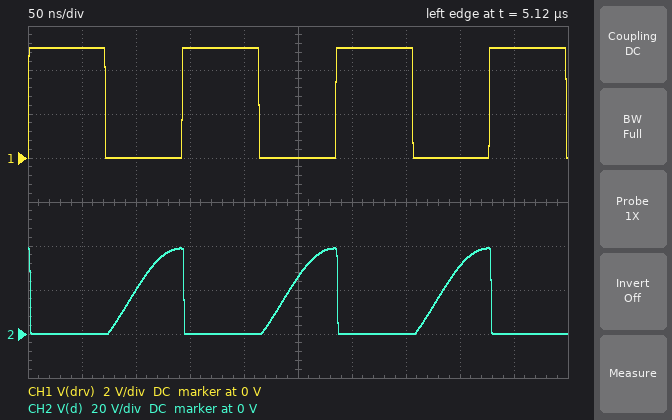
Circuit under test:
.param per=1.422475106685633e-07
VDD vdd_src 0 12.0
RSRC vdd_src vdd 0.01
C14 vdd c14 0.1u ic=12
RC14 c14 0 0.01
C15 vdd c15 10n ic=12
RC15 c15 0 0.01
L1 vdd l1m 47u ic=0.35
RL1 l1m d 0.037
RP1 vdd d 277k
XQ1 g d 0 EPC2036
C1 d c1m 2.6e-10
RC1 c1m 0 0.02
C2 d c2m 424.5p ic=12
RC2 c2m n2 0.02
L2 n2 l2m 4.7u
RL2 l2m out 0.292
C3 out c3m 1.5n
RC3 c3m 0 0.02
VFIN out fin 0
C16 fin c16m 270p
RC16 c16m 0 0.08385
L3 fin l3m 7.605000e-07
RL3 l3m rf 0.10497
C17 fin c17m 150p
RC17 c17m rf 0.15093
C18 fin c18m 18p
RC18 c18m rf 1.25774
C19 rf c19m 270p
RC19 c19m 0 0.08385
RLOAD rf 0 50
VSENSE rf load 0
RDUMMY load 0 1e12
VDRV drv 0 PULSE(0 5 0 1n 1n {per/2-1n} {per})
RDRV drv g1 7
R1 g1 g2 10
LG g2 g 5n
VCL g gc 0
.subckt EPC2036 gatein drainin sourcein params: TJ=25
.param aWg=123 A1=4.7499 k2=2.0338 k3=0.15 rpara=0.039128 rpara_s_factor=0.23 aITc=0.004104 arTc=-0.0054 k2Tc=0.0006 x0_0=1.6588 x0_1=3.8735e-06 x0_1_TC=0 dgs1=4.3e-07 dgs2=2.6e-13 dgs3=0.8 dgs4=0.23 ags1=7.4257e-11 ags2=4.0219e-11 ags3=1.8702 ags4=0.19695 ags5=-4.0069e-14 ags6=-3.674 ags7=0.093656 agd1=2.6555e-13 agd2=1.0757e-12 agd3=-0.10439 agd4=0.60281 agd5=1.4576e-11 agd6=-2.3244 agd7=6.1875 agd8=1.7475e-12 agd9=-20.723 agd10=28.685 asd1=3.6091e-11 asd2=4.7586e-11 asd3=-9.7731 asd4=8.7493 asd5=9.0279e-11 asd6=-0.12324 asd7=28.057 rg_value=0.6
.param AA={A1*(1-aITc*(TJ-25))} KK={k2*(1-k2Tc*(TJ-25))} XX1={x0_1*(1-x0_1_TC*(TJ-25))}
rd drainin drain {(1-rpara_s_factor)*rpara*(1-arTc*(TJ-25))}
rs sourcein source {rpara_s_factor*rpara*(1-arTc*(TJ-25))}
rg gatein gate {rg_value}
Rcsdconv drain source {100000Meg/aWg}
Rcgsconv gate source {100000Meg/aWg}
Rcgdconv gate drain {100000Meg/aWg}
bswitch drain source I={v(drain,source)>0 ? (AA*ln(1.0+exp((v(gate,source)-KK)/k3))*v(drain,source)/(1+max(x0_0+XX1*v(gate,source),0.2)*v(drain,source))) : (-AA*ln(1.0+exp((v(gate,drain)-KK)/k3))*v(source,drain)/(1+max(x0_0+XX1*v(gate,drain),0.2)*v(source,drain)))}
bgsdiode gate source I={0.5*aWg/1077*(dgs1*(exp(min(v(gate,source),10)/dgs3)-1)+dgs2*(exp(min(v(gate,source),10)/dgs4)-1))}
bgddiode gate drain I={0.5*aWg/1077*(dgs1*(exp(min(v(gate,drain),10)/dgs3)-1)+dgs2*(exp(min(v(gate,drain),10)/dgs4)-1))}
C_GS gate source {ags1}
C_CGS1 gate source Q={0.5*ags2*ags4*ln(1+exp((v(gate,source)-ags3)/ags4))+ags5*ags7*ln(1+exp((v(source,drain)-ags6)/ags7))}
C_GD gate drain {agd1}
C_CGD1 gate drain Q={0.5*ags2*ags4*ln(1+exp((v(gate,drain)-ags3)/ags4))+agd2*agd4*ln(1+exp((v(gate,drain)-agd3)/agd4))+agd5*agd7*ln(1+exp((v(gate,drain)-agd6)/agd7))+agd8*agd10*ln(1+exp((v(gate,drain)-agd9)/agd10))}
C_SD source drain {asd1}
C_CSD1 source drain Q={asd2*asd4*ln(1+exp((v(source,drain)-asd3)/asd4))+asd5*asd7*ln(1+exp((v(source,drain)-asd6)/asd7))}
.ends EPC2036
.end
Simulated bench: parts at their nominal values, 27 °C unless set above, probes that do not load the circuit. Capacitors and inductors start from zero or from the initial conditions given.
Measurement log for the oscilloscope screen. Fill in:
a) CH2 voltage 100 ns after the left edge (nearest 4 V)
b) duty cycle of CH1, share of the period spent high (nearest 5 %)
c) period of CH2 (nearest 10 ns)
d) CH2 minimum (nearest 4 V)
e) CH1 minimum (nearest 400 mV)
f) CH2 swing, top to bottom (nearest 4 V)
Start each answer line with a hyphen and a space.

- 20 V
- 50 %
- 140 ns
- 0 V
- 0 V
- 40 V
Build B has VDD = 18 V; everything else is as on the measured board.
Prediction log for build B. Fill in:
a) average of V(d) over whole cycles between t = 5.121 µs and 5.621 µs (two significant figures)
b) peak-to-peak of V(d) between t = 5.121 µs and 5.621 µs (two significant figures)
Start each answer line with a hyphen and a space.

- 18 V
- 58 V
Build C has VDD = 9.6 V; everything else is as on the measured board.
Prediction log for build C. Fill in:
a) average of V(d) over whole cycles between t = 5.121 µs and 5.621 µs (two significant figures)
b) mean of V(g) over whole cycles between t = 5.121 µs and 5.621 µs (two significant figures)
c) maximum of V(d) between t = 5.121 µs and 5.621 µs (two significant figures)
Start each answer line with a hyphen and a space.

- 9.6 V
- 2.5 V
- 31 V
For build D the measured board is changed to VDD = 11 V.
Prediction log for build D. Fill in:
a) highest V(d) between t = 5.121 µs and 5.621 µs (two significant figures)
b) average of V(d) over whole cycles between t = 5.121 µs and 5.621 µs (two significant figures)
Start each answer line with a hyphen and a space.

- 36 V
- 11 V
